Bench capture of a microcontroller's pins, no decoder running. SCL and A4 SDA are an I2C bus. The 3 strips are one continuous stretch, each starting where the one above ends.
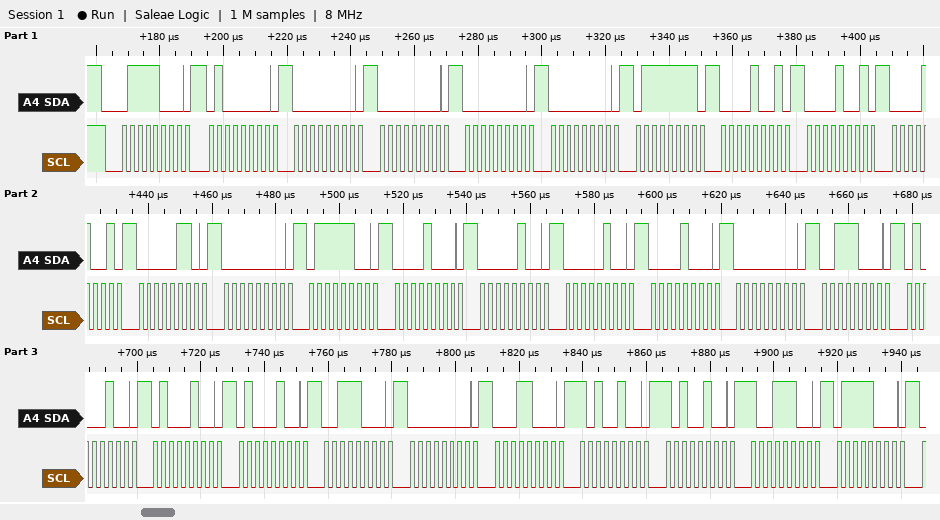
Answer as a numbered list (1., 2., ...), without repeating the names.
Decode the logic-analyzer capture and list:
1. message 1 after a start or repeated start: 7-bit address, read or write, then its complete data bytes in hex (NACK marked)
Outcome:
1. 0x3C write: 40 00 00 00 00 7F 09 09 09 06 00 7C 08 04 04 08 00 38 44 44 44 38 00 18 A4 A4 9C 78
